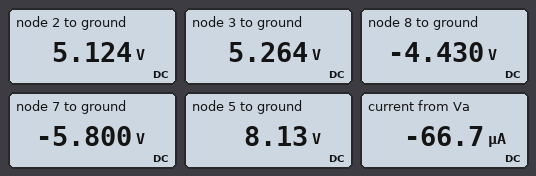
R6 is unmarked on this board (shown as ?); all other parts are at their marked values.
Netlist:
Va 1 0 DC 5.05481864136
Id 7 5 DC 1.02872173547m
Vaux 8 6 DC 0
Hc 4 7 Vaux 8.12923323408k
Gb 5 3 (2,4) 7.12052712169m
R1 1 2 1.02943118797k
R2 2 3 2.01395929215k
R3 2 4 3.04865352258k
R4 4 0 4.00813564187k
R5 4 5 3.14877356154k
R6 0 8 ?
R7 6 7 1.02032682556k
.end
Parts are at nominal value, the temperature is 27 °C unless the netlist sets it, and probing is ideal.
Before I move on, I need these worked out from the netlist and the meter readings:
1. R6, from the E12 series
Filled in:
3.3 kΩ
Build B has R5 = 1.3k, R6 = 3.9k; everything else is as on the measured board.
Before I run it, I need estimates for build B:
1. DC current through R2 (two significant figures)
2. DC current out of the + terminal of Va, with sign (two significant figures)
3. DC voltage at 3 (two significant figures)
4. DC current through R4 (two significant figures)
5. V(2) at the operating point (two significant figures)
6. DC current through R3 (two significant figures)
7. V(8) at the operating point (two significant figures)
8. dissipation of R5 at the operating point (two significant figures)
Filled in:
350 µA
-330 µA
6.1 V
1.3 mA
5.4 V
16 µA
-6.5 V
600 µW
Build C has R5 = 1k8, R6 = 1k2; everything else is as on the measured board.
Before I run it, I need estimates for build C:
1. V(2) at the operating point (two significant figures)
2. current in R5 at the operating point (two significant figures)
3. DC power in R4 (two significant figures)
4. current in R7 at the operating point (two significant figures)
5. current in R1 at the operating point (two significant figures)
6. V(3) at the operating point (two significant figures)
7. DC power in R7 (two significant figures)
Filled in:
4.7 V
1.4 mA
5.6 mW
800 µA
380 µA
3.9 V
650 µW
